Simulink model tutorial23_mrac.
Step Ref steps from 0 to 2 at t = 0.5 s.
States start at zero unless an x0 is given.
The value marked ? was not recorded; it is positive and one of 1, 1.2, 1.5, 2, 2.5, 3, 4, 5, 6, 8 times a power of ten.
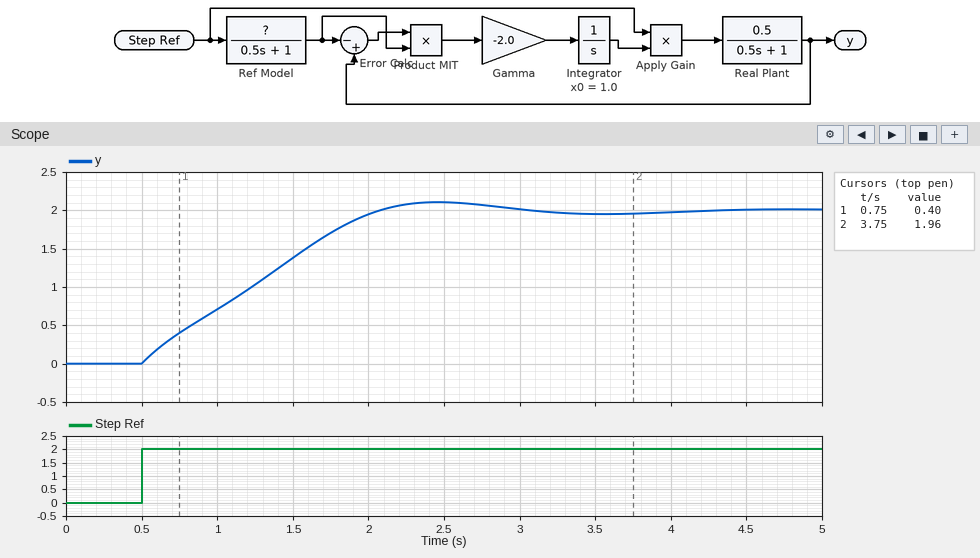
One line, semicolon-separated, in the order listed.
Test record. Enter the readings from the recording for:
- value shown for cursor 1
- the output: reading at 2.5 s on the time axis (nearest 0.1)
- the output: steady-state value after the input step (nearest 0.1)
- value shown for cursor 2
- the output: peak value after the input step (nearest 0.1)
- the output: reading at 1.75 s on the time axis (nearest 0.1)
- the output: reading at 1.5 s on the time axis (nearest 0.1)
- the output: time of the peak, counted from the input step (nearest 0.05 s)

0.40; 2.1; 2.0; 1.96; 2.1; 1.7; 1.4; 1.95 s
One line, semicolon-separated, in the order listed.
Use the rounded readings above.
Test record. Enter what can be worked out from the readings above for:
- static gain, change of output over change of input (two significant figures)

1.0
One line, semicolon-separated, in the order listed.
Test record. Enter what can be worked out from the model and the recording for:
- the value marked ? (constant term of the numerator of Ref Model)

1
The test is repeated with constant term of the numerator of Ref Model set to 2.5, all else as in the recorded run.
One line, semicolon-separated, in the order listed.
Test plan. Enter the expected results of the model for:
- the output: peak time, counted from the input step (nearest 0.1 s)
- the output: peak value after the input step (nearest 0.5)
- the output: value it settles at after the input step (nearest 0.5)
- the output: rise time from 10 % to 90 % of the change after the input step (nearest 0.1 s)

1.3 s; 5.5; 5.0; 0.7 s
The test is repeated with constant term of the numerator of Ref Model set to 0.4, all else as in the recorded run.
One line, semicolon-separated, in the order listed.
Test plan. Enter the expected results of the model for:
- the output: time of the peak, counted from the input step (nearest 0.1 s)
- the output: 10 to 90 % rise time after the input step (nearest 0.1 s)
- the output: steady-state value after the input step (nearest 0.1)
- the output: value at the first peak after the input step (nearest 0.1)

1.3 s; 0.6 s; 0.8; 0.8
